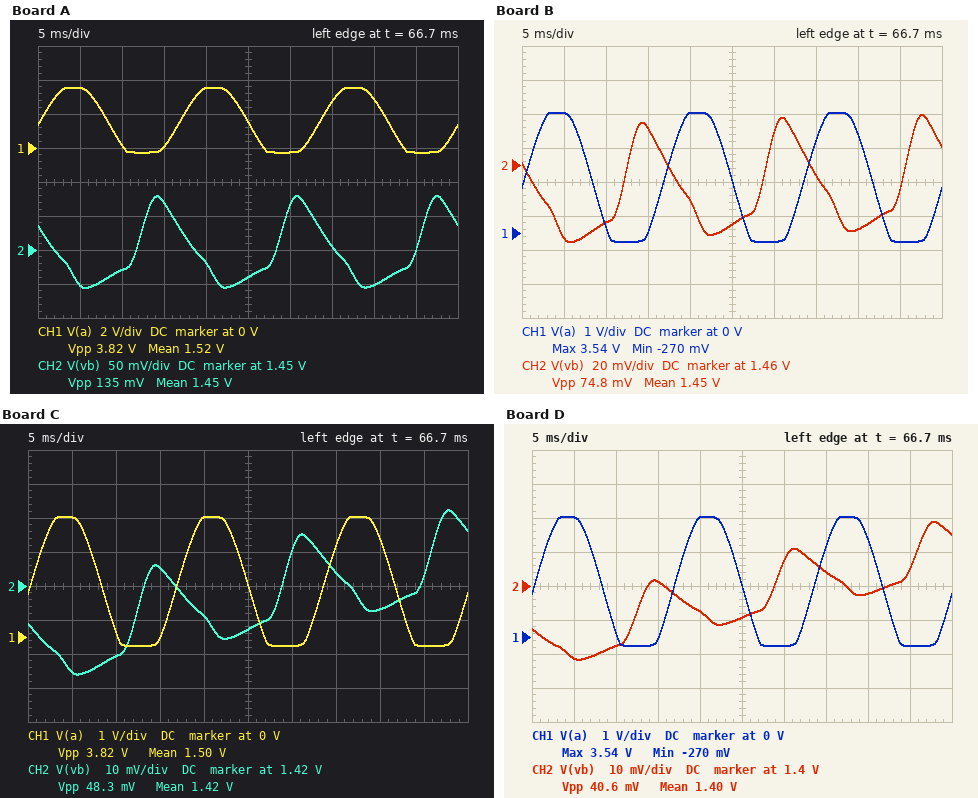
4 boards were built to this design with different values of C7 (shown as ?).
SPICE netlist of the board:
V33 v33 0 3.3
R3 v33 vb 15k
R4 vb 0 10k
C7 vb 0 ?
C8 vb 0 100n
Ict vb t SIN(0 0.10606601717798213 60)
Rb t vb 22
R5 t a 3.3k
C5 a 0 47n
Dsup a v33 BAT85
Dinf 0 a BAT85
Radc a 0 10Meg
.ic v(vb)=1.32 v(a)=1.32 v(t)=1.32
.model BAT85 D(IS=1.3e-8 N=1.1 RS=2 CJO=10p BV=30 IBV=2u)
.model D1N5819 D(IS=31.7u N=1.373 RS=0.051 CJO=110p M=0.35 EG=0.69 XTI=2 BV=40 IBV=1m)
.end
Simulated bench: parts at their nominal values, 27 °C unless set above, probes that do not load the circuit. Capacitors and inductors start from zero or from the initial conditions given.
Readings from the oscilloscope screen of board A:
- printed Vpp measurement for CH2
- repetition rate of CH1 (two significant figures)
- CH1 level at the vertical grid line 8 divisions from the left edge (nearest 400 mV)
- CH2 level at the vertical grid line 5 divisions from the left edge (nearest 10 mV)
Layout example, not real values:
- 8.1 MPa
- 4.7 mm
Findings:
- 135 mV
- 60 Hz
- 2.8 V
- 1.41 V
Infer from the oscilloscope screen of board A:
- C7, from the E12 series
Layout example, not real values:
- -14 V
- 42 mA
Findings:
- 3.3 µF
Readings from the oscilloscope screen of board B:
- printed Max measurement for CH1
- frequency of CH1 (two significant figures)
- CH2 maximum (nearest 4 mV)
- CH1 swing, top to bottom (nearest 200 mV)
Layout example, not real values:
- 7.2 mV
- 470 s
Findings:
- 3.54 V
- 60 Hz
- 1.488 V
- 3.8 V
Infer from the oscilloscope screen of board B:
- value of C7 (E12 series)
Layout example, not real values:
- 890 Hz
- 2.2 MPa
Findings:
- 6.8 µF
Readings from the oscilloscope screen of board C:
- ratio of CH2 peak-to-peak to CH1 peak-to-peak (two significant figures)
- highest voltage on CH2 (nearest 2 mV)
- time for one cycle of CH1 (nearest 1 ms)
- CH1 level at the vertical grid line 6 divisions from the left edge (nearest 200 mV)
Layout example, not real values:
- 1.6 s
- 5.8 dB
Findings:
- 0.013
- 1.442 V
- 17 ms
- -200 mV
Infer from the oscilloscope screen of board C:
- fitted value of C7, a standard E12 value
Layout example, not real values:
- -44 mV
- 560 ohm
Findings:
- 18 µF
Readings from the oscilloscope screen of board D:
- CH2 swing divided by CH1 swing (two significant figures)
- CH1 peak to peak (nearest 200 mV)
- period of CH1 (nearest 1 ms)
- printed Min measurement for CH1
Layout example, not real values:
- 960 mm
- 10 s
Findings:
- 0.011
- 3.8 V
- 17 ms
- -270 mV
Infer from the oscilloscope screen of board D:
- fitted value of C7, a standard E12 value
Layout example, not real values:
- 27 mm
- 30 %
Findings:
- 27 µF
